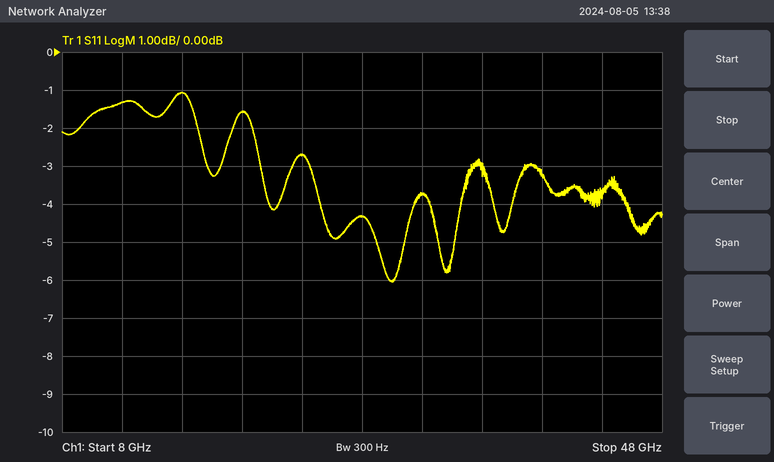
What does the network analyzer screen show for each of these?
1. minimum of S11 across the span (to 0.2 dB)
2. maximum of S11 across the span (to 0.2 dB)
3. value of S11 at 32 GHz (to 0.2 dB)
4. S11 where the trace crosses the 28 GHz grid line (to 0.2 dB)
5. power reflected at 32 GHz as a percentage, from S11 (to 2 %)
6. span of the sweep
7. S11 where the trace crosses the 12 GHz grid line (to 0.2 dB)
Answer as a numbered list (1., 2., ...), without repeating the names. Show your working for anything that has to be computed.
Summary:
1. -6.0 dB
2. -1.0 dB
3. -3.8 dB
4. -4.4 dB
5. 10^(-3.8/10) ≈ 42 %
6. 40 GHz
7. -1.4 dB
